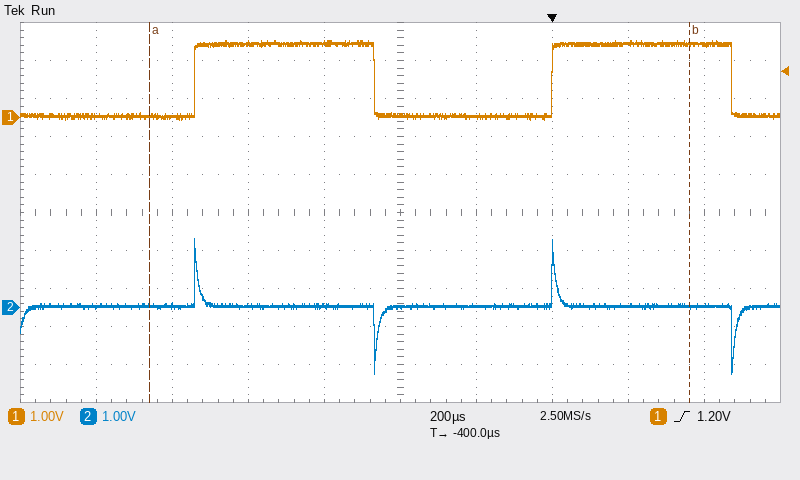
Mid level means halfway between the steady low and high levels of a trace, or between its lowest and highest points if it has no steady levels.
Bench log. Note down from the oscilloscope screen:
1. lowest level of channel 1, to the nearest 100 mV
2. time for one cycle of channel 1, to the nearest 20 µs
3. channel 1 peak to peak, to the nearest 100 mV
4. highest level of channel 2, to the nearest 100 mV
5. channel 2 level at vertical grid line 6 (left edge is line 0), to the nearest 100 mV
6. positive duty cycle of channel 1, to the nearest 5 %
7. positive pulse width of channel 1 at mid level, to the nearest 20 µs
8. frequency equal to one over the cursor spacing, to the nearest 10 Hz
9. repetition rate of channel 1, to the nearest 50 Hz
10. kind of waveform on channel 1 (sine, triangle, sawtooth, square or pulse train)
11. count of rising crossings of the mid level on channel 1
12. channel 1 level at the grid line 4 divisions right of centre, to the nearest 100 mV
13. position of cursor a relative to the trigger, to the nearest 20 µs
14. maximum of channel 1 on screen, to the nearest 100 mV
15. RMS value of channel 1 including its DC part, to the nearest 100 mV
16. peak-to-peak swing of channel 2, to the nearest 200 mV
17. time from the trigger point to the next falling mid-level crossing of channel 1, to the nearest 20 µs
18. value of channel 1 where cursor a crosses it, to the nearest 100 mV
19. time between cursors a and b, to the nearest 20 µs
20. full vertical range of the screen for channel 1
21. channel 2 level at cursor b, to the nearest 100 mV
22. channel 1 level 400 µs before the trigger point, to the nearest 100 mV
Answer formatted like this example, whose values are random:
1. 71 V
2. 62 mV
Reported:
1. -100 mV
2. 940 µs
3. 2.1 V
4. 1.8 V
5. 100 mV
6. 50 %
7. 480 µs
8. 700 Hz
9. 1.05 kHz
10. square
11. 2
12. 1.9 V
13. -1.06 ms
14. 2.0 V
15. 1.4 V
16. 3.6 V
17. 480 µs
18. 100 mV
19. 1.42 ms
20. 10 V
21. 0.0 V
22. 100 mV
